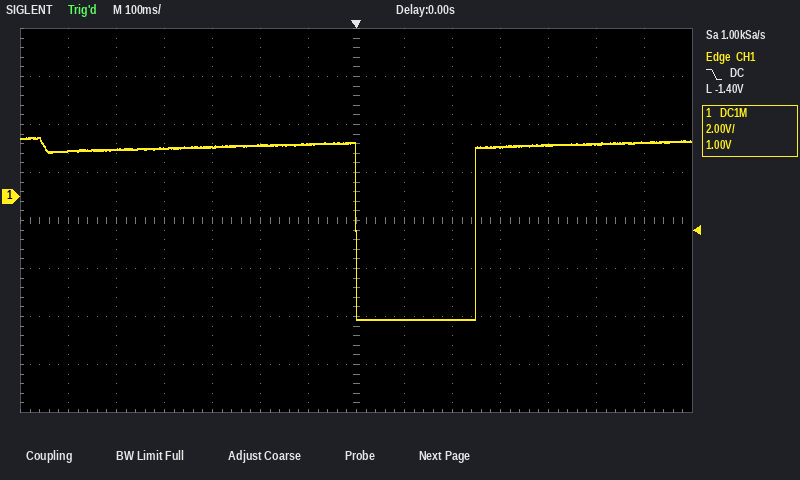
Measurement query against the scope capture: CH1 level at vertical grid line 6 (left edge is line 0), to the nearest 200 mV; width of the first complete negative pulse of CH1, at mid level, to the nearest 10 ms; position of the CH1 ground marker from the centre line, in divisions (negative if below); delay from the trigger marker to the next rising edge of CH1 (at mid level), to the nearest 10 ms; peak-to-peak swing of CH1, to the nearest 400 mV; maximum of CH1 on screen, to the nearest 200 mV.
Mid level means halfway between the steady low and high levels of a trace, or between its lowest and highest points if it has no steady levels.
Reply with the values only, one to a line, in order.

2.2 V
250 ms
+0.5 div
250 ms
7.6 V
2.4 V
